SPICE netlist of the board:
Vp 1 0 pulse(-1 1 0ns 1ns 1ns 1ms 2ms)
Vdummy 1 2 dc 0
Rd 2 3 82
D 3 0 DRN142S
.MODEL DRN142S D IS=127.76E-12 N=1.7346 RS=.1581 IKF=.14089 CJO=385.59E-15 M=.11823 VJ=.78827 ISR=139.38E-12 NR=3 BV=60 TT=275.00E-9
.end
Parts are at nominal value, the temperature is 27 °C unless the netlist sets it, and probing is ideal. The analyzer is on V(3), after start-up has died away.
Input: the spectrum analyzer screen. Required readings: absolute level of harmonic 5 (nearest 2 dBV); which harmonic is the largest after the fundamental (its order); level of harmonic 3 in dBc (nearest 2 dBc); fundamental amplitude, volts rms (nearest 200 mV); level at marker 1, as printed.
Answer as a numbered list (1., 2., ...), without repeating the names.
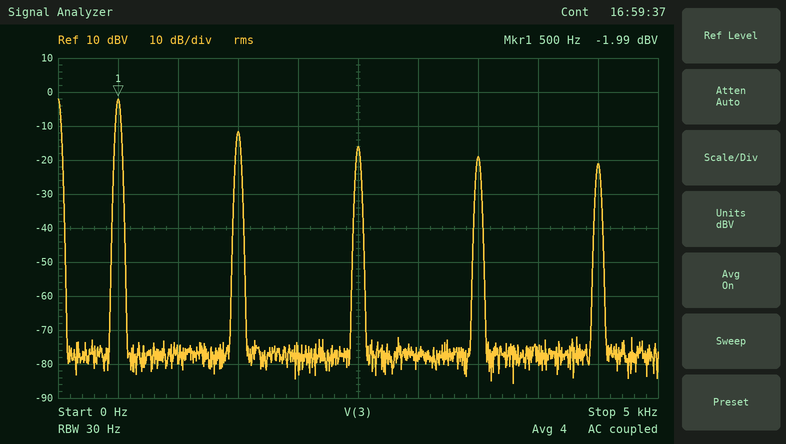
1. -16 dBV
2. 3
3. -10 dBc
4. 800 mV
5. -1.99 dBV
